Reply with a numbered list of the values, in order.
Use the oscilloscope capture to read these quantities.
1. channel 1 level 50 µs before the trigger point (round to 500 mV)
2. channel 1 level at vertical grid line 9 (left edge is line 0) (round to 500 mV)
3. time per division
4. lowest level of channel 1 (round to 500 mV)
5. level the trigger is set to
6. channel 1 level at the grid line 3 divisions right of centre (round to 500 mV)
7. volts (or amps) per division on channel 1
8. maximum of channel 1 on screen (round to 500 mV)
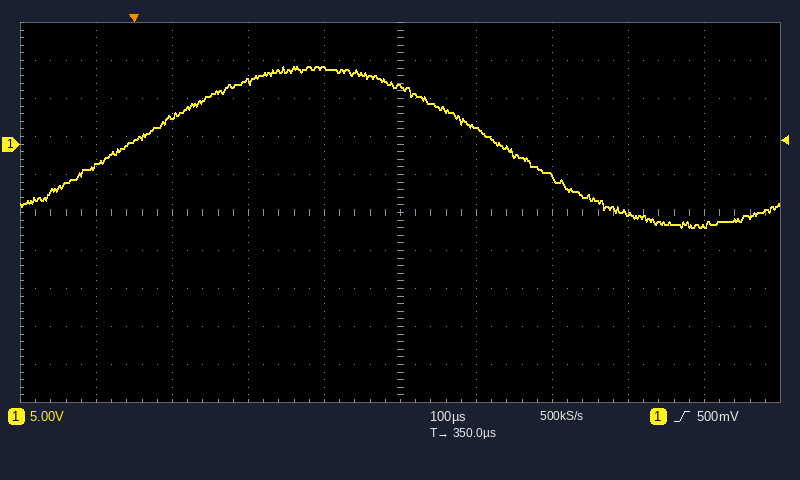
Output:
1. -3.0 V
2. -10.5 V
3. 100 µs
4. -11.0 V
5. 500 mV
6. -9.0 V
7. 5 V
8. 10.0 V
